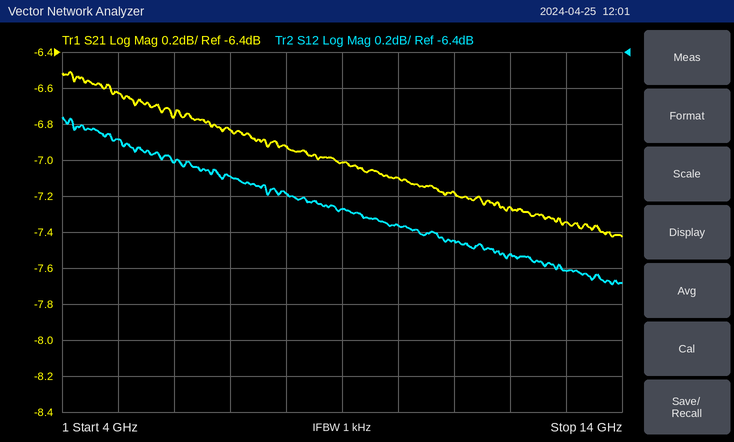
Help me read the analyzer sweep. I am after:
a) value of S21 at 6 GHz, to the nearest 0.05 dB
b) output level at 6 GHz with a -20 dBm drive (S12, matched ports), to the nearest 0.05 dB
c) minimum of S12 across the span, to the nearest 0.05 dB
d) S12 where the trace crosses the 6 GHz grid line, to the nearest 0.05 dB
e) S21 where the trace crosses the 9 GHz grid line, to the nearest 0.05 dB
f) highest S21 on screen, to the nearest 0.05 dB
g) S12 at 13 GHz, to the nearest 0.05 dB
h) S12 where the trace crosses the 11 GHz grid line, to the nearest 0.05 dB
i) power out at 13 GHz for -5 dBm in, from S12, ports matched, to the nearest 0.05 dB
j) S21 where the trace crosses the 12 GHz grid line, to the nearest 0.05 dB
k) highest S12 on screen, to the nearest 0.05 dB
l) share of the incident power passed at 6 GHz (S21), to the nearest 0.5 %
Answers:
-6.75 dB
-27.00 dBm
-7.70 dB
-7.00 dB
-7.00 dB
-6.50 dB
-7.60 dB
-7.45 dB
-12.60 dBm
-7.25 dB
-6.75 dB
21.0 %
